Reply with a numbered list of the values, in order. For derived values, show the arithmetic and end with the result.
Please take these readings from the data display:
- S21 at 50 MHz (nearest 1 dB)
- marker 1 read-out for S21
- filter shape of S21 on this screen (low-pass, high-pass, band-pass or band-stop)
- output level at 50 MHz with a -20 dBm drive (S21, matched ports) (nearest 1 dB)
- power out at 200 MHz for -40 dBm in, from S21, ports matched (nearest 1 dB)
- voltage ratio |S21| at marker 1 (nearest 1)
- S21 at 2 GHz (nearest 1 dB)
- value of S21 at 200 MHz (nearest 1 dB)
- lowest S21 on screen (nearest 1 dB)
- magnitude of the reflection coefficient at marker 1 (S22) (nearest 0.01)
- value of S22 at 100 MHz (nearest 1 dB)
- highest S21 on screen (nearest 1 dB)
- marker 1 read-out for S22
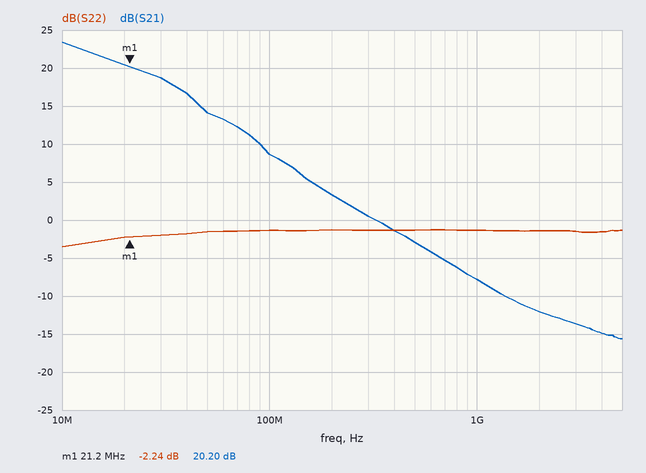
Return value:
1. 14 dB
2. 20.20 dB
3. low-pass
4. -20 dBm + (14 dB) = -6 dBm
5. -40 dBm + (3 dB) = -37 dBm
6. 10^(20.2/20) ≈ 10
7. -12 dB
8. 3 dB
9. -16 dB
10. 10^(-2.24/20) ≈ 0.77
11. -1 dB
12. 23 dB
13. -2.24 dB
